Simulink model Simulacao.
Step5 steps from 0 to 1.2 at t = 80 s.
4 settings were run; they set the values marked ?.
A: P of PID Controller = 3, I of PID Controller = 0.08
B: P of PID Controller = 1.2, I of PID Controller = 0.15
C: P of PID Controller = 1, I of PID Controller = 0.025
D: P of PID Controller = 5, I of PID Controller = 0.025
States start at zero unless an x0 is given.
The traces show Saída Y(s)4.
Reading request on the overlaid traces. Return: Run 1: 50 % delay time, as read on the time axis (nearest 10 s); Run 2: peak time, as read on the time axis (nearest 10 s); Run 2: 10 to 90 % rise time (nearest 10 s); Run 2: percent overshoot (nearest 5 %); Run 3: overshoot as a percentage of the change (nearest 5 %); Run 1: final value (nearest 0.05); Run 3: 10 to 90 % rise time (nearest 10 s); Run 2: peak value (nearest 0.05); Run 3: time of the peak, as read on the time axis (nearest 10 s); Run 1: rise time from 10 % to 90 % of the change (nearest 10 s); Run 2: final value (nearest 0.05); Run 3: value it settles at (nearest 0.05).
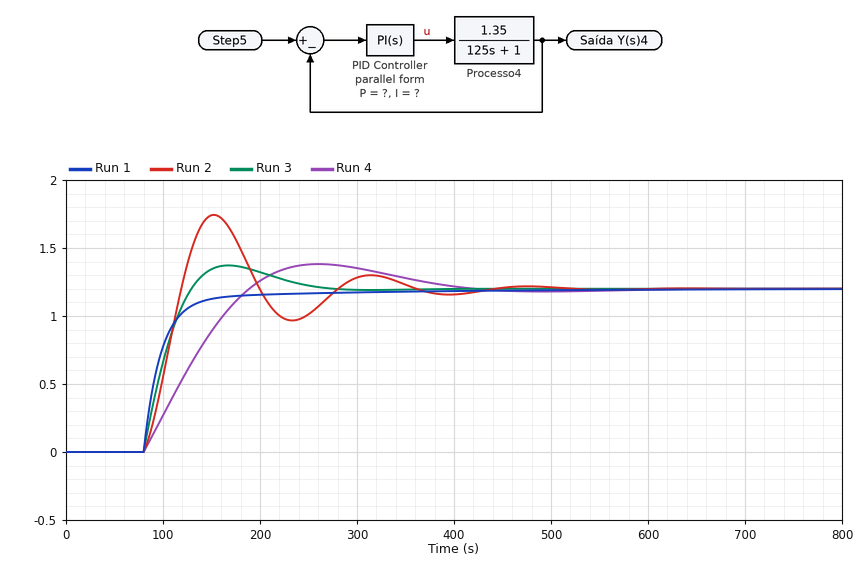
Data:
90 s
150 s
30 s
45 %
15 %
1.20
40 s
1.75
170 s
50 s
1.20
1.20
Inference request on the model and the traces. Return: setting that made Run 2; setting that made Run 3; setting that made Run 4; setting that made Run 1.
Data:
B
A
C
D
